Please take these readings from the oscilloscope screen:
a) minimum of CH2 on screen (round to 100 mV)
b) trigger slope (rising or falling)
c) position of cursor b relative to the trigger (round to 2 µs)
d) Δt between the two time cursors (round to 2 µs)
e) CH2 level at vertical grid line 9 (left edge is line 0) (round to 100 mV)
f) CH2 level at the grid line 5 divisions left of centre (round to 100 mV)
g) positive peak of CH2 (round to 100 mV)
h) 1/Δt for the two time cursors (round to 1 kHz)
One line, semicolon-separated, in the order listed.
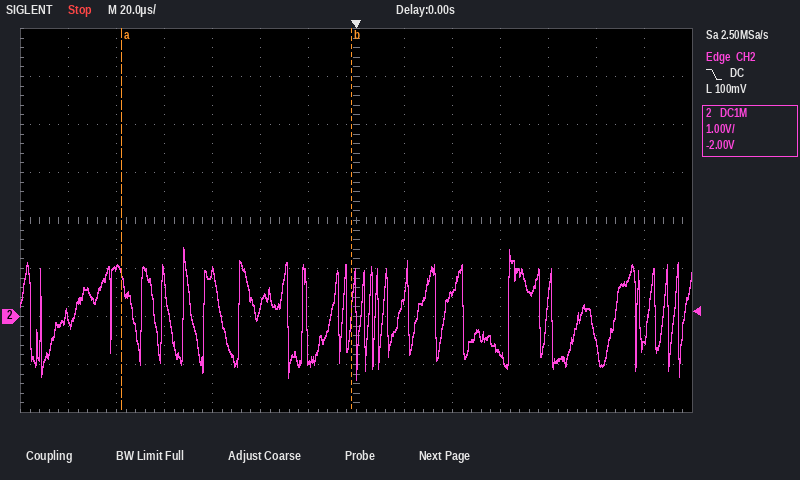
-1.3 V; falling; -2 µs; 96 µs; 500 mV; 1.0 V; 1.4 V; 10 kHz
